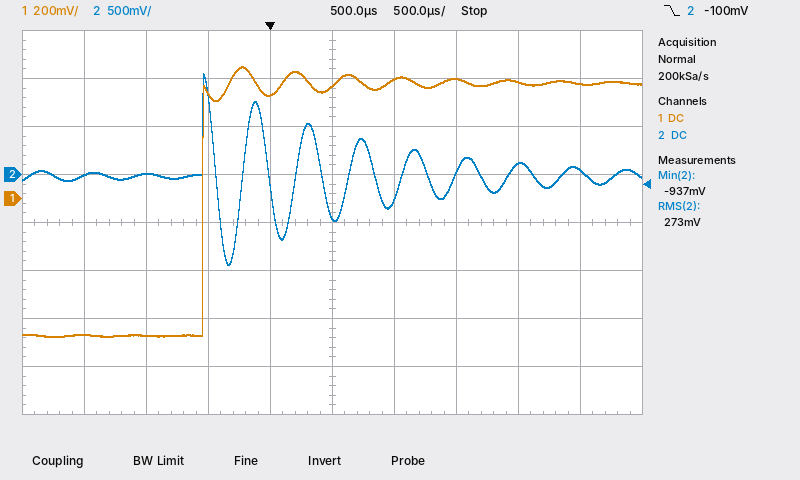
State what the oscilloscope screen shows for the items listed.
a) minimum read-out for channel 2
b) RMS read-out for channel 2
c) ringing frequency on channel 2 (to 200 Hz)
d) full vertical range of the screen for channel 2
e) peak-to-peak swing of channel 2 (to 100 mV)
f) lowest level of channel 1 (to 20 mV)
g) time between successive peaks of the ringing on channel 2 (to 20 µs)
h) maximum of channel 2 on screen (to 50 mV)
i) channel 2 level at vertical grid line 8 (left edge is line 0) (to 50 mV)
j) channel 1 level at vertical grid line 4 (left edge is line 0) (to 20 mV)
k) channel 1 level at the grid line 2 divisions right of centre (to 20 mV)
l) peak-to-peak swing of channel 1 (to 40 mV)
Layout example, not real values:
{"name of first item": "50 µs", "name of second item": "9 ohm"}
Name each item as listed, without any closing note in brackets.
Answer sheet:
{"minimum read-out for channel 2": "-937 mV", "RMS read-out for channel 2": "273 mV", "ringing frequency on channel 2": "2.4 kHz", "full vertical range of the screen for channel 2": "4 V", "peak-to-peak swing of channel 2": "2.00 V", "lowest level of channel 1": "-580 mV", "time between successive peaks of the ringing on channel 2": "420 µs", "maximum of channel 2 on screen": "1.05 V", "channel 2 level at vertical grid line 8 (left edge is line 0)": "100 mV", "channel 1 level at vertical grid line 4 (left edge is line 0)": "440 mV", "channel 1 level at the grid line 2 divisions right of centre": "500 mV", "peak-to-peak swing of channel 1": "1.12 V"}
